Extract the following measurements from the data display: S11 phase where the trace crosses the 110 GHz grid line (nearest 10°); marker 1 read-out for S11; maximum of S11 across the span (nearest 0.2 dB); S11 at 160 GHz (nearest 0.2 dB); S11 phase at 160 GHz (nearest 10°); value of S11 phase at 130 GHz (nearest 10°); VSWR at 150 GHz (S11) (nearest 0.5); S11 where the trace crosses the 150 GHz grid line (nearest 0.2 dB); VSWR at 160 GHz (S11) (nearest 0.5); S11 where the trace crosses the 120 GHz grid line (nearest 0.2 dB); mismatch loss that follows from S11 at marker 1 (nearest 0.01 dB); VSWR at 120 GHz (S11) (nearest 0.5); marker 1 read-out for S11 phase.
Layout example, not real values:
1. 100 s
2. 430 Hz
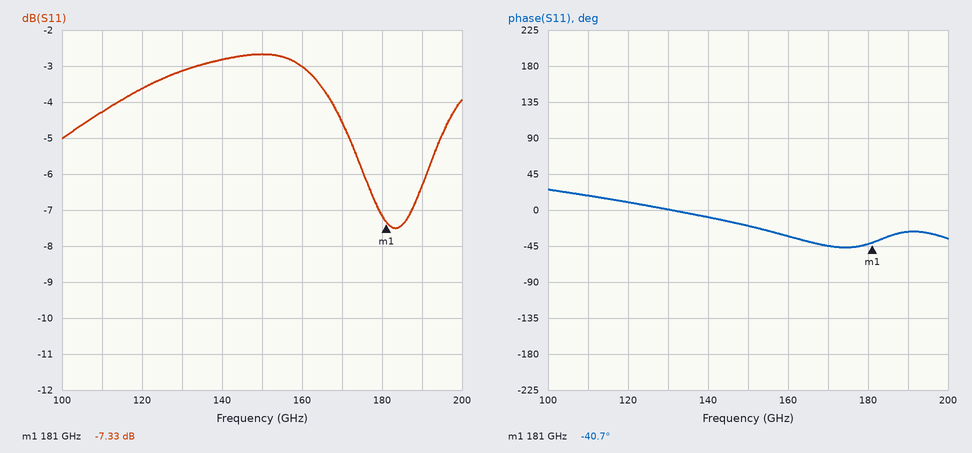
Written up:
1. 20°
2. -7.33 dB
3. -2.6 dB
4. -3.0 dB
5. -30°
6. 0°
7. 6.5
8. -2.6 dB
9. 6.0
10. -3.6 dB
11. 0.89 dB
12. 5.0
13. -40.7°
